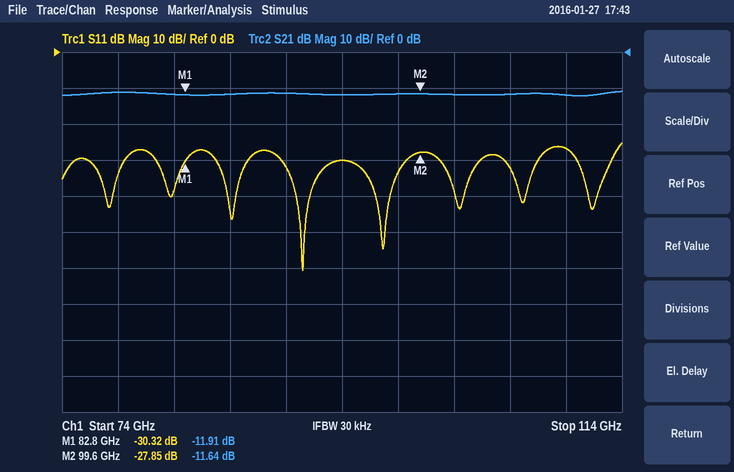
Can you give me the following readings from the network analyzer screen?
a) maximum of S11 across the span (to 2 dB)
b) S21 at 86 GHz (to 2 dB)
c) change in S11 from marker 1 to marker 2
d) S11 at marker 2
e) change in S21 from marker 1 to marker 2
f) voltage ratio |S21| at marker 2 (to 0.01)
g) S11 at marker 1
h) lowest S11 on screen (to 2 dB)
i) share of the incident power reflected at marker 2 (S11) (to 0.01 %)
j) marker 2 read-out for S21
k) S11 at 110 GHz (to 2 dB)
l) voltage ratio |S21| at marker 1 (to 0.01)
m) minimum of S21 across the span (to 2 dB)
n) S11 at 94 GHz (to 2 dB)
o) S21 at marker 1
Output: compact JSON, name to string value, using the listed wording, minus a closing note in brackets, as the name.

{"maximum of S11 across the span": "-26 dB", "S21 at 86 GHz": "-12 dB", "change in S11 from marker 1 to marker 2": "2.47 dB", "S11 at marker 2": "-27.85 dB", "change in S21 from marker 1 to marker 2": "0.27 dB", "voltage ratio |S21| at marker 2": "0.26", "S11 at marker 1": "-30.32 dB", "lowest S11 on screen": "-60 dB", "share of the incident power reflected at marker 2 (S11)": "0.16 %", "marker 2 read-out for S21": "-11.64 dB", "S11 at 110 GHz": "-26 dB", "voltage ratio |S21| at marker 1": "0.25", "minimum of S21 across the span": "-12 dB", "S11 at 94 GHz": "-30 dB", "S21 at marker 1": "-11.91 dB"}
